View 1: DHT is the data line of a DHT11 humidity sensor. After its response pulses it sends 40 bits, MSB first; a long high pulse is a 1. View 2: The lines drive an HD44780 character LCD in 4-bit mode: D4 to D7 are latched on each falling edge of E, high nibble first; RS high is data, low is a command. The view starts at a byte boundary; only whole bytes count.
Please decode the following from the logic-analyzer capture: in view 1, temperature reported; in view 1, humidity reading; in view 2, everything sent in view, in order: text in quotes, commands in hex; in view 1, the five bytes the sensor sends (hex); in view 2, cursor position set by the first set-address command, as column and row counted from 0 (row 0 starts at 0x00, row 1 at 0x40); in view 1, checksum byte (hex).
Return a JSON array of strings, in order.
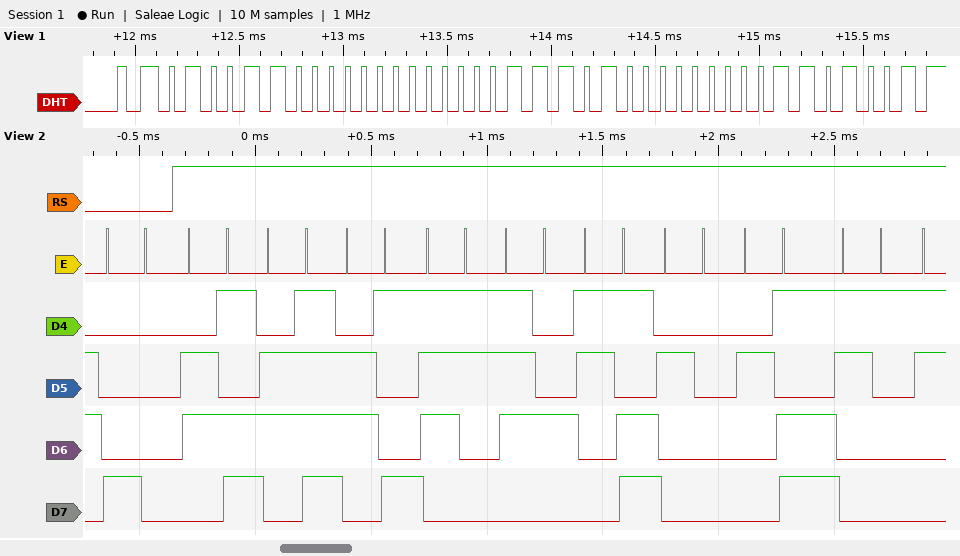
["29.0 °C", "76 %", "0x80 \"moist= -1\"", "4C 00 1D 00 69", "column 0, row 0", "0x69"]
